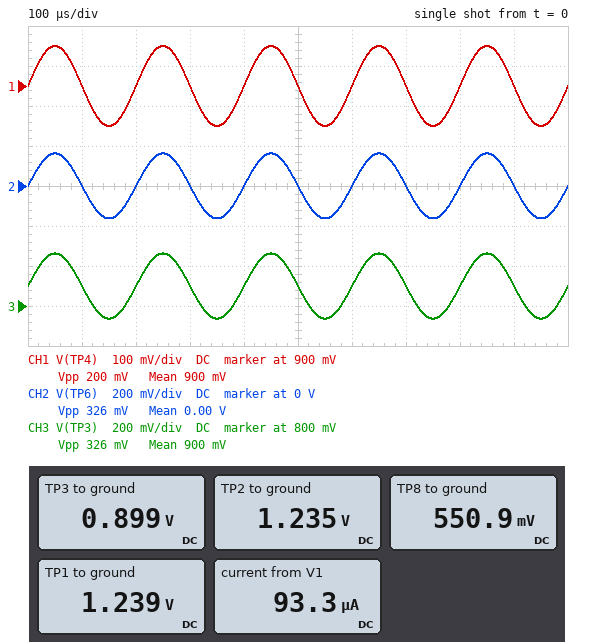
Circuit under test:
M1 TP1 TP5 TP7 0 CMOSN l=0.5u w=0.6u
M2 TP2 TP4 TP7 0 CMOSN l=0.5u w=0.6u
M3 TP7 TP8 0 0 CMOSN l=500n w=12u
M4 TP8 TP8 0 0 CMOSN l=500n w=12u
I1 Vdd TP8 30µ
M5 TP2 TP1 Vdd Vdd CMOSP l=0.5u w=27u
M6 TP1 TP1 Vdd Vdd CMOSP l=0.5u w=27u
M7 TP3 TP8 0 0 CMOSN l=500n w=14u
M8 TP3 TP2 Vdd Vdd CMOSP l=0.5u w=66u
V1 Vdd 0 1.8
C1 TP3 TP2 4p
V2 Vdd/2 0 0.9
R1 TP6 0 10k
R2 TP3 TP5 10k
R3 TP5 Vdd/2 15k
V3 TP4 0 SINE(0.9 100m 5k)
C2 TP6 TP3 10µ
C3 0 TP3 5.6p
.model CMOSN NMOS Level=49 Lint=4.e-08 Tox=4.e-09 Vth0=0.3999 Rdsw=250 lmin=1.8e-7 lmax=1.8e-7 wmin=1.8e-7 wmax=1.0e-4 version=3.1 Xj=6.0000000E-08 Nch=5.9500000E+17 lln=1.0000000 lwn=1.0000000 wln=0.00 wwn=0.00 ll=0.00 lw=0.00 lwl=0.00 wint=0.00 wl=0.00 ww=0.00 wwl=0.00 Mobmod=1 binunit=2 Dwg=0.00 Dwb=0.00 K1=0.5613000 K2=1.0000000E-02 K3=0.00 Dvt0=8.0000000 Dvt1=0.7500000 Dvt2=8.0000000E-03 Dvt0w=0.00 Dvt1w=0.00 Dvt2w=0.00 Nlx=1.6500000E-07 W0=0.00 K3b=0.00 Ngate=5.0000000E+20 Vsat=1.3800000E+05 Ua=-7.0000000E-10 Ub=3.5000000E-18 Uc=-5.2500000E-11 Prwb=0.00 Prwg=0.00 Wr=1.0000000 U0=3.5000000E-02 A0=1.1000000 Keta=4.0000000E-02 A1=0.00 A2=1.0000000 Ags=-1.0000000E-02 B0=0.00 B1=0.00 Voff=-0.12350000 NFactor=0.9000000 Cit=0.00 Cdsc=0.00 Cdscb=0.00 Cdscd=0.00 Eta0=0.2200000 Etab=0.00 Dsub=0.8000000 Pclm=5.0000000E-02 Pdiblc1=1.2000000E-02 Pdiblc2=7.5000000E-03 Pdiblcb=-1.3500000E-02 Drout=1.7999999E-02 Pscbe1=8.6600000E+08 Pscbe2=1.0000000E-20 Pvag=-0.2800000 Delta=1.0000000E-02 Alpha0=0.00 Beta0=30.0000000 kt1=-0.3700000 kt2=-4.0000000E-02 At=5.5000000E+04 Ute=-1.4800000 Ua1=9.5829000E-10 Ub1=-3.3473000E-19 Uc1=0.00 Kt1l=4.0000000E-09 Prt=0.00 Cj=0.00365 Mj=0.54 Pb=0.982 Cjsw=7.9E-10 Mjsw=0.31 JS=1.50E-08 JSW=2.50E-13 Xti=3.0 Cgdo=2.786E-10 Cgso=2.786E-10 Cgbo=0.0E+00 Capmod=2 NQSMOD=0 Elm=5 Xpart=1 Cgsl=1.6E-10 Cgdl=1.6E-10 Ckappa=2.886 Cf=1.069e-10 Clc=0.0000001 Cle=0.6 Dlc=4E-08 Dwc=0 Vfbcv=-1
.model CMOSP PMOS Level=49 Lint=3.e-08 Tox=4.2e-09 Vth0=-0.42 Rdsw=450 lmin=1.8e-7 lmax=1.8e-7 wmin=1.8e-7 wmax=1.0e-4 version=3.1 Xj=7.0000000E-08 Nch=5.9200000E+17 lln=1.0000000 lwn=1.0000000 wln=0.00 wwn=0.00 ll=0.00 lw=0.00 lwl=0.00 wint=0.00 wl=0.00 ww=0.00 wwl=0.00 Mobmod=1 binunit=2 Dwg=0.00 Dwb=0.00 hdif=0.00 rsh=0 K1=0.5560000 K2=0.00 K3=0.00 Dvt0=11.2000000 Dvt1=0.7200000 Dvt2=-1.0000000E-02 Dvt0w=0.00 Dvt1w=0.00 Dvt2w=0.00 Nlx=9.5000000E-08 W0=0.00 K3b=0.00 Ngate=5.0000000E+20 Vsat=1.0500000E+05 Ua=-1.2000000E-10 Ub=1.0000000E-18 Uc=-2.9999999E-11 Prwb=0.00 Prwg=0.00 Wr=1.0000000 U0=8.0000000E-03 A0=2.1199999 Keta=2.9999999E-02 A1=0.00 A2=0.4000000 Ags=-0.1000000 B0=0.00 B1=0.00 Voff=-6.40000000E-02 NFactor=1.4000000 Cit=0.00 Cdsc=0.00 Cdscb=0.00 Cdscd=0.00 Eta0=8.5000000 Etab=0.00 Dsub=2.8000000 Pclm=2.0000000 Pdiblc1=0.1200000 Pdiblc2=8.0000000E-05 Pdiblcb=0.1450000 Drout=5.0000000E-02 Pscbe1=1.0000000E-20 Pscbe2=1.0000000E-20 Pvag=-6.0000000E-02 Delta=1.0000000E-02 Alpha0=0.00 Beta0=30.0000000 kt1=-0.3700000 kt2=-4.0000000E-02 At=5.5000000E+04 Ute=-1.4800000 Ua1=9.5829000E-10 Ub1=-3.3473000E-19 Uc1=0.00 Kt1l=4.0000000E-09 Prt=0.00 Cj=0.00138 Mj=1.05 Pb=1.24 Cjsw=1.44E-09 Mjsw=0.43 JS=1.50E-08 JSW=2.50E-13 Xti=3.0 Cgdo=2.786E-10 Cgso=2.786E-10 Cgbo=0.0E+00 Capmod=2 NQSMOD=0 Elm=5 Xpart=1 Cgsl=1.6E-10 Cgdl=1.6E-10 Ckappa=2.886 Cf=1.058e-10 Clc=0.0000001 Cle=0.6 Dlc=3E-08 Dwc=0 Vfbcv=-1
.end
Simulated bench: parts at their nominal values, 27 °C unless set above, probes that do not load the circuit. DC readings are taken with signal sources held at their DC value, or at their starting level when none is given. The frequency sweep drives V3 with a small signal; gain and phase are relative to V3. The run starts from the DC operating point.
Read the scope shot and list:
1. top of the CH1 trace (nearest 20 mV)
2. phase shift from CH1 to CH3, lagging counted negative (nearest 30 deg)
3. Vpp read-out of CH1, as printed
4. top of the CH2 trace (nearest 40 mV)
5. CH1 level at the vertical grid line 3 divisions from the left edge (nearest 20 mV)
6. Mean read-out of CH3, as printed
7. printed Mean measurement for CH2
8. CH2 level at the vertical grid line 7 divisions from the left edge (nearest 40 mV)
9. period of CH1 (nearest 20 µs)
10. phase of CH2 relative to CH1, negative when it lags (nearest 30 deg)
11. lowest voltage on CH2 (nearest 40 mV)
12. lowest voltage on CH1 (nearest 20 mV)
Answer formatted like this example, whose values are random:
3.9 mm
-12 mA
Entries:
1.00 V
0 deg
200 mV
160 mV
900 mV
900 mV
0.00 V
0 V
200 µs
0 deg
-160 mV
800 mV
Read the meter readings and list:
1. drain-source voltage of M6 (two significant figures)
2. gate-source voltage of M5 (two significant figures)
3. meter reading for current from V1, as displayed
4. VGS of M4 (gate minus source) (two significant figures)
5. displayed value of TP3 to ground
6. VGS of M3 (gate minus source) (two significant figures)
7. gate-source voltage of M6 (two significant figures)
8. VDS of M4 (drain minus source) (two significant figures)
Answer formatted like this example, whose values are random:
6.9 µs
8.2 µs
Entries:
-560 mV
-560 mV
93.3 µA
550 mV
0.899 V
550 mV
-560 mV
550 mV
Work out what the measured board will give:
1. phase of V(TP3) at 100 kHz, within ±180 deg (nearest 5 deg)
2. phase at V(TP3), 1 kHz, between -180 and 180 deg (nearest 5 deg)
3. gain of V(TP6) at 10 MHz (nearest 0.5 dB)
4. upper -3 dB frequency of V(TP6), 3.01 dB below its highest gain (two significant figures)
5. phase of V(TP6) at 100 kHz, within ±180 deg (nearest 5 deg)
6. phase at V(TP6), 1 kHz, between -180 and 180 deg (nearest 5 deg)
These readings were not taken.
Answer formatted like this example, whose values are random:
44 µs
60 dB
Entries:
-5 deg
0 deg
-12.0 dB
1.7 MHz
-5 deg
0 deg
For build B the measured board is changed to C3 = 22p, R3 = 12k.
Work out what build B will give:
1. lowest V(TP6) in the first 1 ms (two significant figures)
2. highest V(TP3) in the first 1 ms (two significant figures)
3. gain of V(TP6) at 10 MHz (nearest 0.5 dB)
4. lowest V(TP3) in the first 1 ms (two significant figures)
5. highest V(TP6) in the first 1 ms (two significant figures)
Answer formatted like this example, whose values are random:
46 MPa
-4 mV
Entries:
-180 mV
1.1 V
-17.5 dB
720 mV
180 mV
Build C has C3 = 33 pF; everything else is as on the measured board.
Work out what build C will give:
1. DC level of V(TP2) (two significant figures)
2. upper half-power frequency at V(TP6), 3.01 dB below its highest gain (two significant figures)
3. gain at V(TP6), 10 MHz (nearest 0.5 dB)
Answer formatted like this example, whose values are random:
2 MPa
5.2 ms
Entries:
1.2 V
2.1 MHz
-20.5 dB
